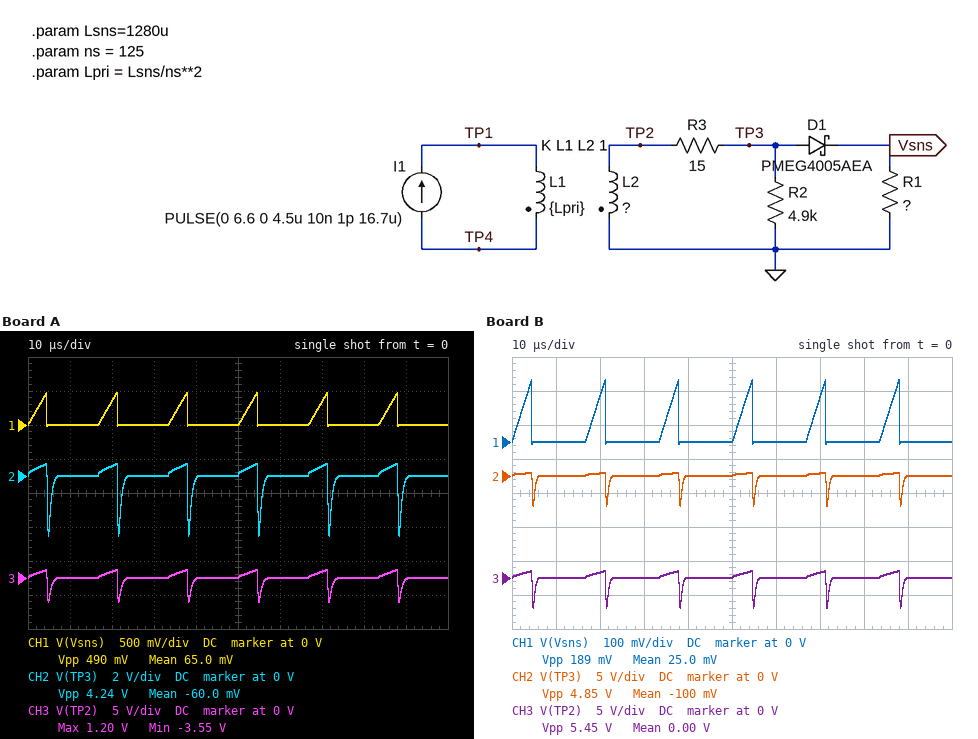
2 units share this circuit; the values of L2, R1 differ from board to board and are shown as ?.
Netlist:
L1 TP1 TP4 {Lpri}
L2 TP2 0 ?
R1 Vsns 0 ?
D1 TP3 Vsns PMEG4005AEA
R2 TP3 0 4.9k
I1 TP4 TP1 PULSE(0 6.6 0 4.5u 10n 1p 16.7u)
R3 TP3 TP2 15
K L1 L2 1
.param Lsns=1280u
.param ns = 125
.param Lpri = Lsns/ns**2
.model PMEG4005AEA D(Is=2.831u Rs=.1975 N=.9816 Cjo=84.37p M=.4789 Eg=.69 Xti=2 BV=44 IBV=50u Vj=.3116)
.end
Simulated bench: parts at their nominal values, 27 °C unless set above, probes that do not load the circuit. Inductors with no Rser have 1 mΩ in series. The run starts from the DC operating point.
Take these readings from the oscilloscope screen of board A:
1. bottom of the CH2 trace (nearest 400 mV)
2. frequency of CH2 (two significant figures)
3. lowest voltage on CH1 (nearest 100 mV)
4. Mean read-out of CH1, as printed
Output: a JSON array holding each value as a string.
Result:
["-3.6 V", "60 kHz", "0 V", "65.0 mV"]
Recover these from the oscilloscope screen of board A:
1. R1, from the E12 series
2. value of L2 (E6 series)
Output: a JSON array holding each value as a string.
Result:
["15 Ω", "3.3 mH"]
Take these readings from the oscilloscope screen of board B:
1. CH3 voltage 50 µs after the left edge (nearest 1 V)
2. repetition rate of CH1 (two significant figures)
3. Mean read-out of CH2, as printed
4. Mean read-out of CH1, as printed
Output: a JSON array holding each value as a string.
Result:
["0 V", "60 kHz", "-100 mV", "25.0 mV"]
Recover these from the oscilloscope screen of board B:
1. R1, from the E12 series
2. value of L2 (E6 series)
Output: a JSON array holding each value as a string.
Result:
["4.7 Ω", "2.2 mH"]
